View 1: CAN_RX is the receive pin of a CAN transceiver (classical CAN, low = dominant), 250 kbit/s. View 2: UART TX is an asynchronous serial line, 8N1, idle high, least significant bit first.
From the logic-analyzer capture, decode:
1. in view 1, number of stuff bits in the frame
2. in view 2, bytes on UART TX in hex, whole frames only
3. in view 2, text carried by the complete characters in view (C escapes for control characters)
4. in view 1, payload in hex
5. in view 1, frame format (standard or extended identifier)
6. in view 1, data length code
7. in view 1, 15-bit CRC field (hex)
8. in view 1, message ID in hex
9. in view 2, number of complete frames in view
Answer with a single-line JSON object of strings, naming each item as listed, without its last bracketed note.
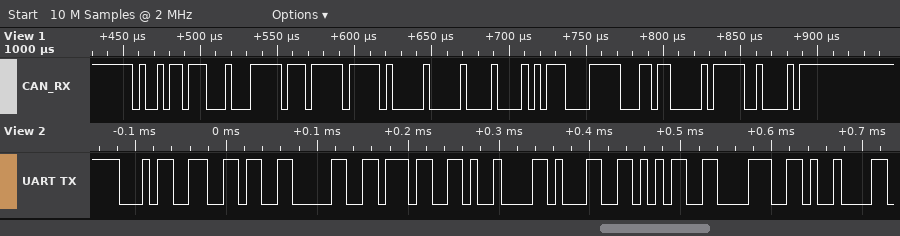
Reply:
{"in view 1, number of stuff bits in the frame": "8", "in view 2, bytes on UART TX in hex, whole frames only": "34 36 30 37 09 31 35 38 09", "in view 2, text carried by the complete characters in view": "\"4607\\t158\\t\"", "in view 1, payload in hex": "FF 7F F0 00 21 5C 3E 6C", "in view 1, frame format": "standard", "in view 1, data length code": "8", "in view 1, 15-bit CRC field": "0x07D0", "in view 1, message ID in hex": "0x4B7", "in view 2, number of complete frames in view": "9"}
